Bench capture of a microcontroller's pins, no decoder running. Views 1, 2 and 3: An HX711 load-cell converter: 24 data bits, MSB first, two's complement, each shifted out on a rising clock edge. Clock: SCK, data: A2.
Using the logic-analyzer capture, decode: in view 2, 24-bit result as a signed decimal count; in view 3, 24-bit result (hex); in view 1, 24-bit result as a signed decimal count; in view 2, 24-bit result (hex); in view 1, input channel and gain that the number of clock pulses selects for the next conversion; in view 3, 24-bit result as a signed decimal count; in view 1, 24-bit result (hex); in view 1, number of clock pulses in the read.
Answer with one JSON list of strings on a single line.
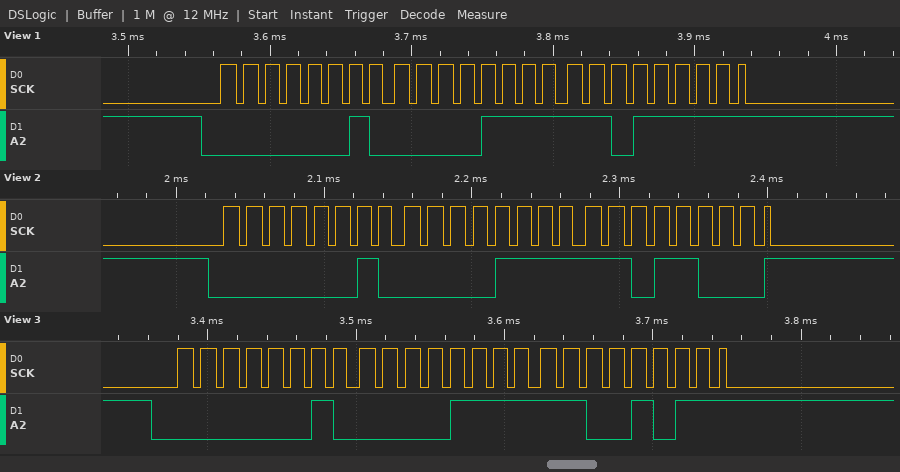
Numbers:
["135128", "0x020FCB", "135135", "0x020FD8", "channel A, gain 128", "135115", "0x020FDF", "25"]
